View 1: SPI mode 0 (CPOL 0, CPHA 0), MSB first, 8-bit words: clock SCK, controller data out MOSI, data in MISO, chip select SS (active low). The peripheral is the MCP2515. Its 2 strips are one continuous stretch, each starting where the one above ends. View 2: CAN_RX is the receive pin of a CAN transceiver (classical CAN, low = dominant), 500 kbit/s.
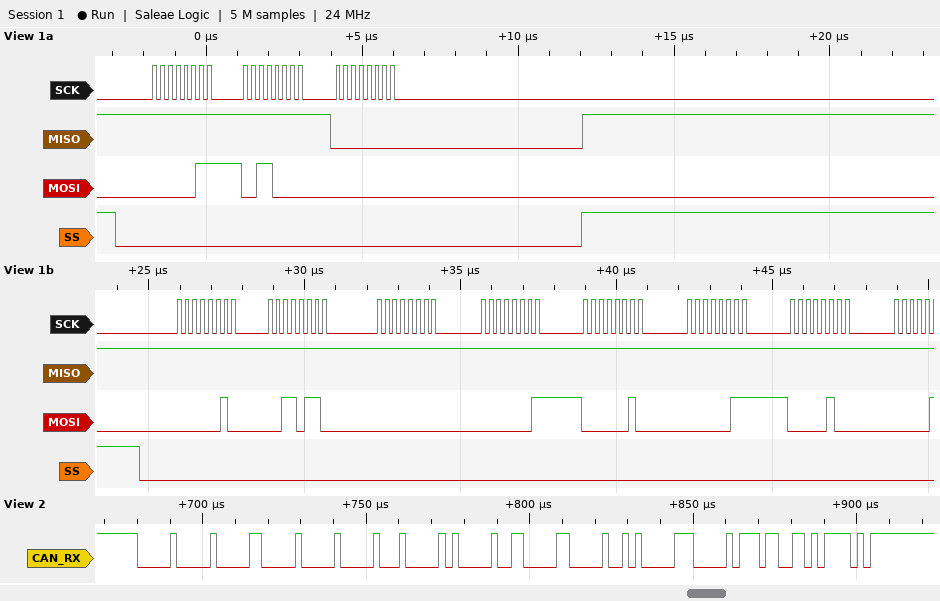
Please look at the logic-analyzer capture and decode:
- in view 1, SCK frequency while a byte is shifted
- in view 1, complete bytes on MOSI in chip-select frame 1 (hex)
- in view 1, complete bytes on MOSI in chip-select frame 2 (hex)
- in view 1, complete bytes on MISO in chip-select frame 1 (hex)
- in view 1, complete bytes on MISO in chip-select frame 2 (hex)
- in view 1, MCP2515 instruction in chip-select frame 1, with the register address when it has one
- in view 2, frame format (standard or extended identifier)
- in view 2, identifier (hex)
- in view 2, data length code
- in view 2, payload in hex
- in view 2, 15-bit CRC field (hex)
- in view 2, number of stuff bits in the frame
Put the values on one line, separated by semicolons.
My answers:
4 MHz; 03 30 00; 02 36 00 01 02 03 04; FF FF 00; FF FF FF FF FF FF FF; READ 0x30; standard; 0x000; 8; 00 01 02 03 04 05 06 07; 0x335E; 12
